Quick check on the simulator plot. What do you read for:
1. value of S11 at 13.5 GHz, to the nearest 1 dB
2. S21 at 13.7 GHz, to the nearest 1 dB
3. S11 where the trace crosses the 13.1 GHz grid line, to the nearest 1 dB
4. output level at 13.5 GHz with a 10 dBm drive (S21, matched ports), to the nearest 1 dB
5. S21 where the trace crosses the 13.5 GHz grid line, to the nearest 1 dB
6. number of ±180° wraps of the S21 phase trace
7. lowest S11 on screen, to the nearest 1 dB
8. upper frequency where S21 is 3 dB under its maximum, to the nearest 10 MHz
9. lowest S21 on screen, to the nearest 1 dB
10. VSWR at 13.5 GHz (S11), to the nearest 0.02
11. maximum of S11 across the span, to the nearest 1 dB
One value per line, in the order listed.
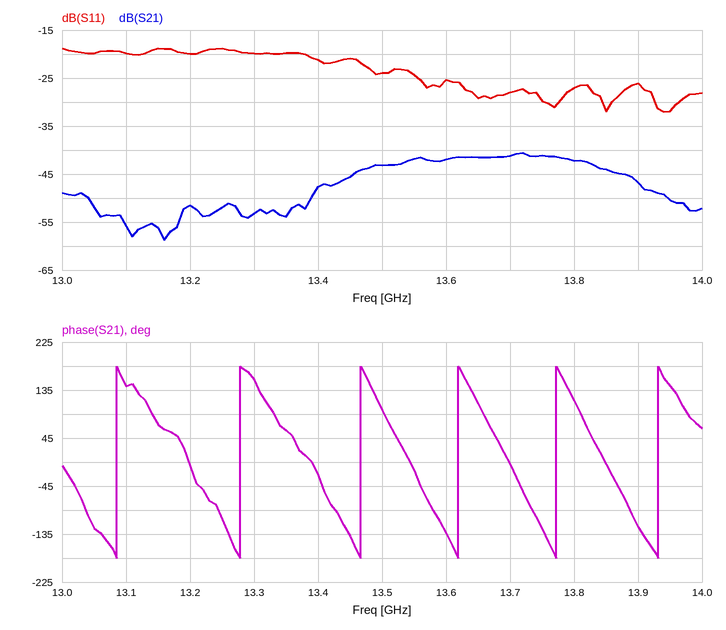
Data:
-24 dB
-41 dB
-20 dB
-33 dBm
-43 dB
6
-32 dB
13.84 GHz
-59 dB
1.14
-19 dB
